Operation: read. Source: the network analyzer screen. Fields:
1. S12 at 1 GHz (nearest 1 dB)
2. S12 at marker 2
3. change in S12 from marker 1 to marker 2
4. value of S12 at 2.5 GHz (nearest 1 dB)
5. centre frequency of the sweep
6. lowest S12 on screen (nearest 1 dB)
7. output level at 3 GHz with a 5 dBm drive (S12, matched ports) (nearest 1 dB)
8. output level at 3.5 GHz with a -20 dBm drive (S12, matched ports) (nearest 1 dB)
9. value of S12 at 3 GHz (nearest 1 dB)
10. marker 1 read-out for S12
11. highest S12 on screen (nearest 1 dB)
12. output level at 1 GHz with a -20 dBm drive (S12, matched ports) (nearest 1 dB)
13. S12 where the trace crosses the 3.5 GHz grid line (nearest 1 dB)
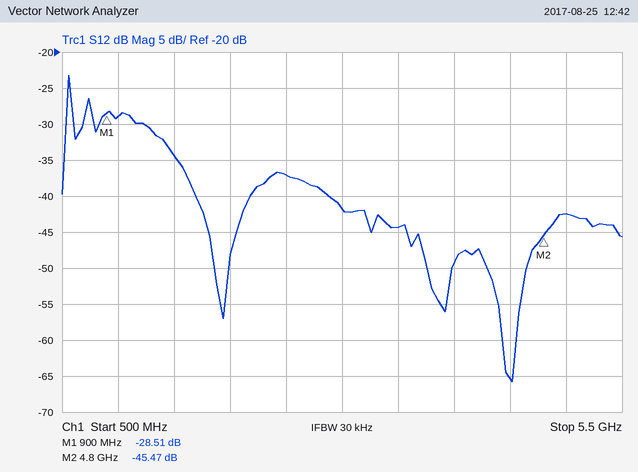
-29 dB
-45.47 dB
-16.96 dB
-37 dB
3 GHz
-66 dB
-37 dBm
-64 dBm
-42 dB
-28.51 dB
-23 dB
-49 dBm
-44 dB
